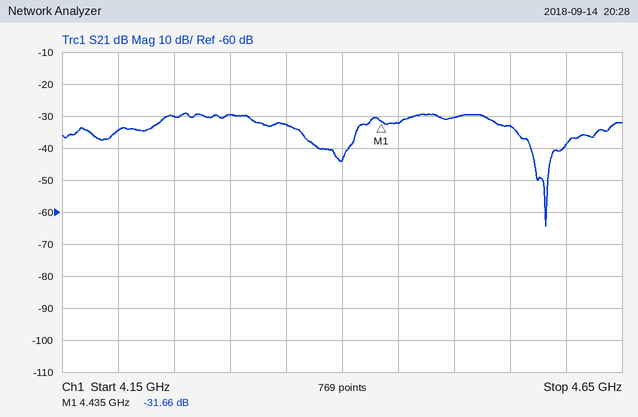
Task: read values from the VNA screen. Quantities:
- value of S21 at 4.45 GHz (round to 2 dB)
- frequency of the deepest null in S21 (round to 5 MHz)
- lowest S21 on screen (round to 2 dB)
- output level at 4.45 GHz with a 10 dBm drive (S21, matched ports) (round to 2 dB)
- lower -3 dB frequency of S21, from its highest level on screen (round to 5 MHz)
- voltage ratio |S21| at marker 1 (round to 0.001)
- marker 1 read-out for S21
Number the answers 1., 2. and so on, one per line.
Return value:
1. -32 dB
2. 4.580 GHz
3. -64 dB
4. -22 dBm
5. 4.235 GHz
6. 0.026
7. -31.66 dB
